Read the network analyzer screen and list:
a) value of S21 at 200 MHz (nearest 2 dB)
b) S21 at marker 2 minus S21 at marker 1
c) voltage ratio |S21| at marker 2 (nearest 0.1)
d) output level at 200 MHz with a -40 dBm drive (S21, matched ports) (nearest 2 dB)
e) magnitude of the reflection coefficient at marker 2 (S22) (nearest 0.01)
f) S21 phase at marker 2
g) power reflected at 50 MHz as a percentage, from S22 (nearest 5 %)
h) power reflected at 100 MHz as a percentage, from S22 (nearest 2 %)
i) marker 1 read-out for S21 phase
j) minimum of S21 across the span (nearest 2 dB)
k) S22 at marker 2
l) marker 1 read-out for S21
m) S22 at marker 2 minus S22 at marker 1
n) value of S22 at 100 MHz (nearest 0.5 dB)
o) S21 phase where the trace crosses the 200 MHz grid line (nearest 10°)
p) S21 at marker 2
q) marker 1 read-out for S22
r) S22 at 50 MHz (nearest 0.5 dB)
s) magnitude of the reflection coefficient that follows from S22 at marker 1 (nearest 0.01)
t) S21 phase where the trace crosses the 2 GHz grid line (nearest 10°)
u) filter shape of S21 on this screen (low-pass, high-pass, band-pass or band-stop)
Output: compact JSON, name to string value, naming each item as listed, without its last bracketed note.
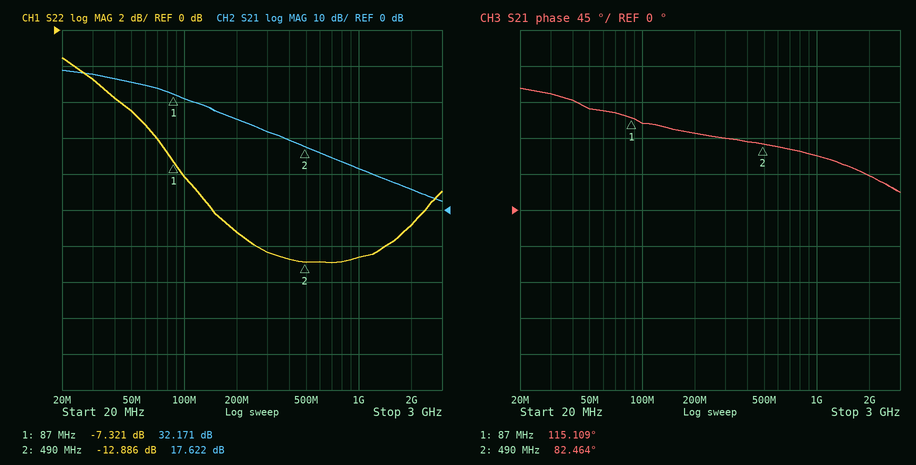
{"value of S21 at 200 MHz": "26 dB", "S21 at marker 2 minus S21 at marker 1": "-14.549 dB", "voltage ratio |S21| at marker 2": "7.6", "output level at 200 MHz with a -40 dBm drive (S21, matched ports)": "-14 dBm", "magnitude of the reflection coefficient at marker 2 (S22)": "0.23", "S21 phase at marker 2": "82.464°", "power reflected at 50 MHz as a percentage, from S22": "35 %", "power reflected at 100 MHz as a percentage, from S22": "16 %", "marker 1 read-out for S21 phase": "115.109°", "minimum of S21 across the span": "2 dB", "S22 at marker 2": "-12.886 dB", "marker 1 read-out for S21": "32.171 dB", "S22 at marker 2 minus S22 at marker 1": "-5.565 dB", "value of S22 at 100 MHz": "-8.0 dB", "S21 phase where the trace crosses the 200 MHz grid line": "100°", "S21 at marker 2": "17.622 dB", "marker 1 read-out for S22": "-7.321 dB", "S22 at 50 MHz": "-4.5 dB", "magnitude of the reflection coefficient that follows from S22 at marker 1": "0.43", "S21 phase where the trace crosses the 2 GHz grid line": "40°", "filter shape of S21 on this screen": "low-pass"}
